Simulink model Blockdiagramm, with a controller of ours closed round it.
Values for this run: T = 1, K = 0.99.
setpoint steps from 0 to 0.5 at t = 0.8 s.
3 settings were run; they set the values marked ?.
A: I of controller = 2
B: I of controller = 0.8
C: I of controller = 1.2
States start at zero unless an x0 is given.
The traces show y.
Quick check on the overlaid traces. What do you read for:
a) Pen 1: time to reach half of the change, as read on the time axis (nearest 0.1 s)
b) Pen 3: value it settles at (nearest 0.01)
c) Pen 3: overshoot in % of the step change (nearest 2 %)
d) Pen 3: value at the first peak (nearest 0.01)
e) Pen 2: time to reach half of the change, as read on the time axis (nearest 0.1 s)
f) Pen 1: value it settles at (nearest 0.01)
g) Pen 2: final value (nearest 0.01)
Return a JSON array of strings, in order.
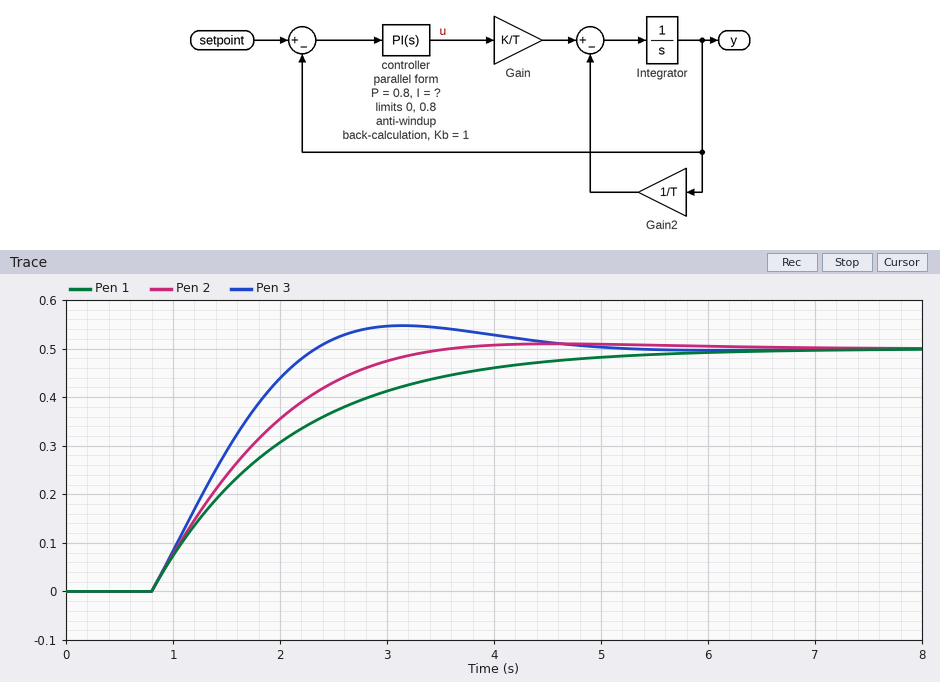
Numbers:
["1.7 s", "0.50", "10 %", "0.55", "1.5 s", "0.50", "0.50"]
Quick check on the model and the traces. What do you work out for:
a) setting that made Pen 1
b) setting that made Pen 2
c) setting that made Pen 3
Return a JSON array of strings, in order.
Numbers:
["B", "C", "A"]
